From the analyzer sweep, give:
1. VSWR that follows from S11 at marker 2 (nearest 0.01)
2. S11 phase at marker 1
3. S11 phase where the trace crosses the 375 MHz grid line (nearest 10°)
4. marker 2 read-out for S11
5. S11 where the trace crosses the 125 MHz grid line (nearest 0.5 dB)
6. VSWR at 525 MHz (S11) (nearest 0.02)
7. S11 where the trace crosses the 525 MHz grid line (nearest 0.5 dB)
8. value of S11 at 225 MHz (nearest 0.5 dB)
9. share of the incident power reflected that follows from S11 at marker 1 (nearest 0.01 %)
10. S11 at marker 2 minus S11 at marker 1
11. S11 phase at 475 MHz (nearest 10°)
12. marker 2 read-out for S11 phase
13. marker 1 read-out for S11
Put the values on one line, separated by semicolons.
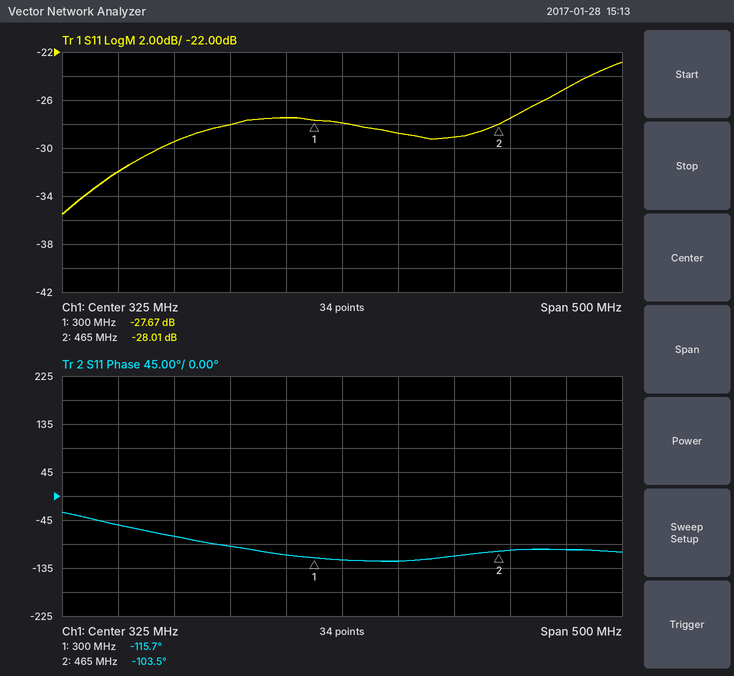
1.08; -115.7°; -120°; -28.01 dB; -32.0 dB; 1.12; -25.0 dB; -28.0 dB; 0.17 %; -0.34 dB; -100°; -103.5°; -27.67 dB
